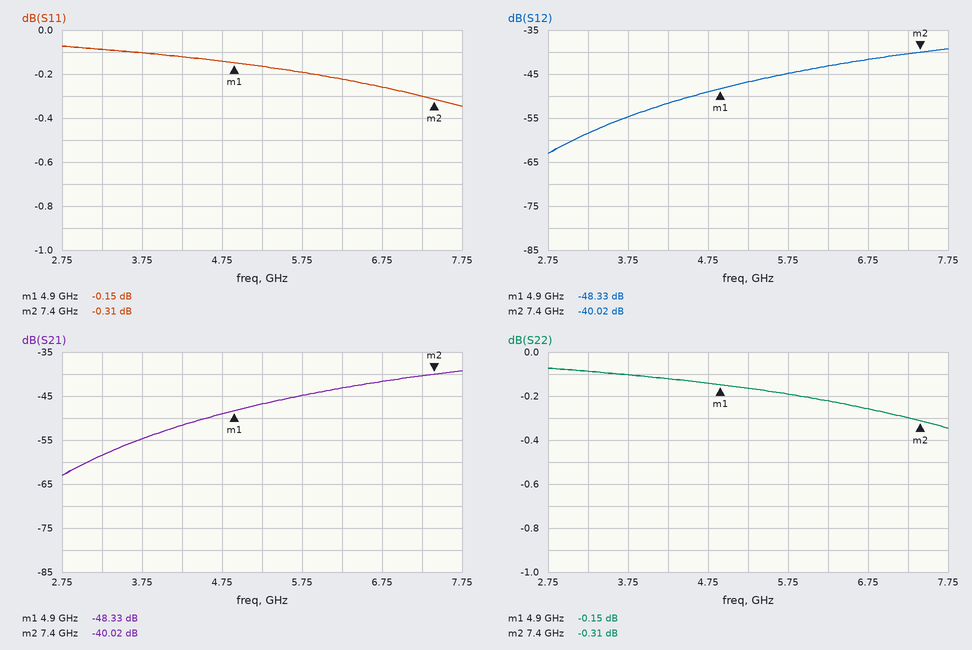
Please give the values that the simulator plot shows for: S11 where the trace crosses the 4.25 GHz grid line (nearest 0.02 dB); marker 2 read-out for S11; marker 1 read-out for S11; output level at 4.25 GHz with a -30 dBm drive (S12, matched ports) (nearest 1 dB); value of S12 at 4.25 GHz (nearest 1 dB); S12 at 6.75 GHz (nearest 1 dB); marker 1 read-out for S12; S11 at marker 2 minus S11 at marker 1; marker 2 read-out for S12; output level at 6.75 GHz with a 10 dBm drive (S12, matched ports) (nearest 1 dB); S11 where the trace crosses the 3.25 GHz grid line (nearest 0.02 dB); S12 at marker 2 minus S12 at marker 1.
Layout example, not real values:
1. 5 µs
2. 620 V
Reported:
1. -0.12 dB
2. -0.31 dB
3. -0.15 dB
4. -82 dBm
5. -52 dB
6. -42 dB
7. -48.33 dB
8. -0.16 dB
9. -40.02 dB
10. -32 dBm
11. -0.08 dB
12. 8.31 dB
